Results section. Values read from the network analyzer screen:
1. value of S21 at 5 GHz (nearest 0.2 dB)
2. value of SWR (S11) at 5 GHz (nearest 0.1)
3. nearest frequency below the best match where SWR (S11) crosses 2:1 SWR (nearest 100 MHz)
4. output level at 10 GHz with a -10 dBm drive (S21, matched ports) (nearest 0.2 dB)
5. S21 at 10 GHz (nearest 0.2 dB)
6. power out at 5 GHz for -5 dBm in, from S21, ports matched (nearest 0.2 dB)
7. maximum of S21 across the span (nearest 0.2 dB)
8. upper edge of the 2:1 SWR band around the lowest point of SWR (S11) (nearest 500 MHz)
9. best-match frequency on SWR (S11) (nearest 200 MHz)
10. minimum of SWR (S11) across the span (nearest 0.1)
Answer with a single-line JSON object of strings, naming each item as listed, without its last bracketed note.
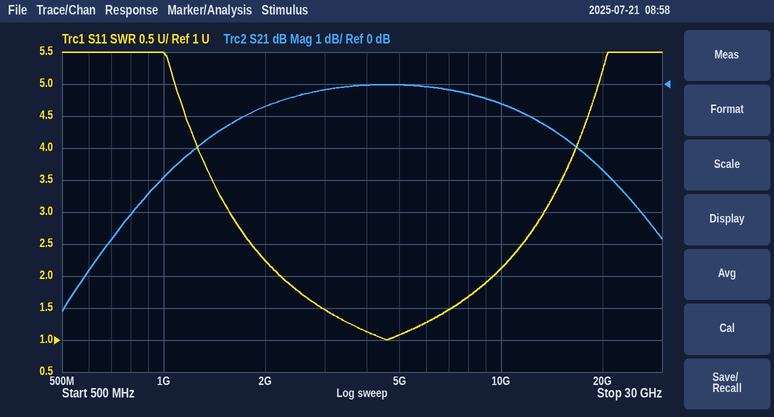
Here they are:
{"value of S21 at 5 GHz": "0.0 dB", "value of SWR (S11) at 5 GHz": "1.1", "nearest frequency below the best match where SWR (S11) crosses 2:1 SWR": "2.2 GHz", "output level at 10 GHz with a -10 dBm drive (S21, matched ports)": "-10.6 dBm", "S21 at 10 GHz": "-0.6 dB", "power out at 5 GHz for -5 dBm in, from S21, ports matched": "-5.0 dBm", "maximum of S21 across the span": "0.0 dB", "upper edge of the 2:1 SWR band around the lowest point of SWR (S11)": "9.5 GHz", "best-match frequency on SWR (S11)": "4.6 GHz", "minimum of SWR (S11) across the span": "1.0"}
